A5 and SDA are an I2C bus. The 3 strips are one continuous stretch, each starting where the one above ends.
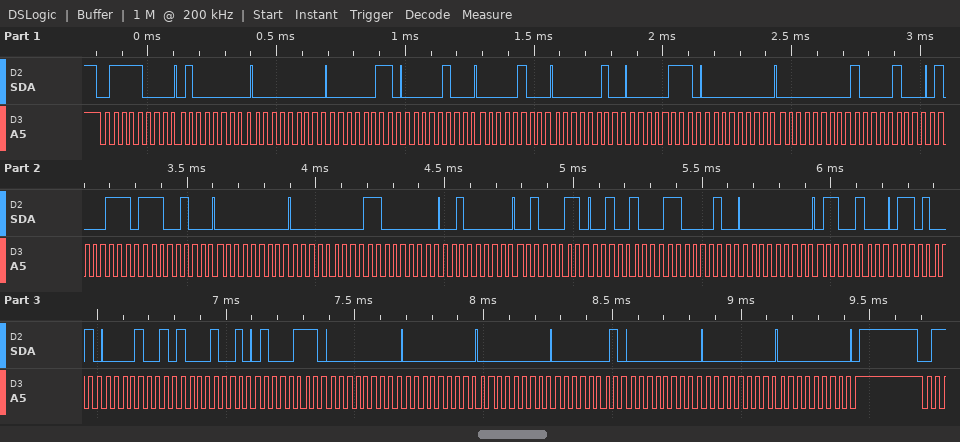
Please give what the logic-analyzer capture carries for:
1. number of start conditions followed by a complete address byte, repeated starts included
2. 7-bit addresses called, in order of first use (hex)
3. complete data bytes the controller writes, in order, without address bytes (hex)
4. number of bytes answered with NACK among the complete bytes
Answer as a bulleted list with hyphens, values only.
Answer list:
- 1
- 0x3C
- 40 00 03 04 04 02 07 00 00 84 47 E4 00 00 C0 20 23 24 C2 00 64 69 09 89 47 00 00 00 01 00 00 00
- 0
